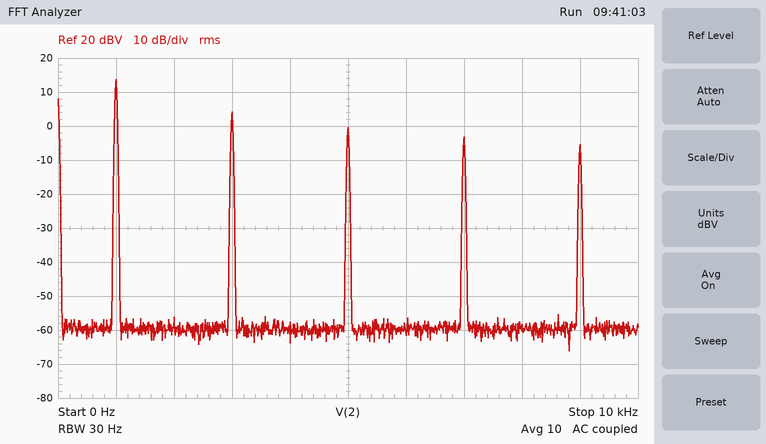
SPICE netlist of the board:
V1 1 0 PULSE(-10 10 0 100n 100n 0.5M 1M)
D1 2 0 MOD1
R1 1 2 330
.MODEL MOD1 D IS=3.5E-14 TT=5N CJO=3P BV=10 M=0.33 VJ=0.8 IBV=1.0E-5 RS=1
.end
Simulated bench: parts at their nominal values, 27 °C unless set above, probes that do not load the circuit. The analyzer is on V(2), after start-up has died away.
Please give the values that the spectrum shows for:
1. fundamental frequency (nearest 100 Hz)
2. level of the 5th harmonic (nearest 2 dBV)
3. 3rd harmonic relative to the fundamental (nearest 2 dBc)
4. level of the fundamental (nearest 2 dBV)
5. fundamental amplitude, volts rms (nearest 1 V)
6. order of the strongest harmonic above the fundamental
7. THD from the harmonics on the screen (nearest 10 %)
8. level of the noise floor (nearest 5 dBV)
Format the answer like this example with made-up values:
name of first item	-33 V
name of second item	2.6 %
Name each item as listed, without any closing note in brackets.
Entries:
fundamental frequency	1.0 kHz
level of the 5th harmonic	0 dBV
3rd harmonic relative to the fundamental	-10 dBc
level of the fundamental	14 dBV
fundamental amplitude, volts rms	5 V
order of the strongest harmonic above the fundamental	3
THD from the harmonics on the screen	40 %
level of the noise floor	-60 dBV
